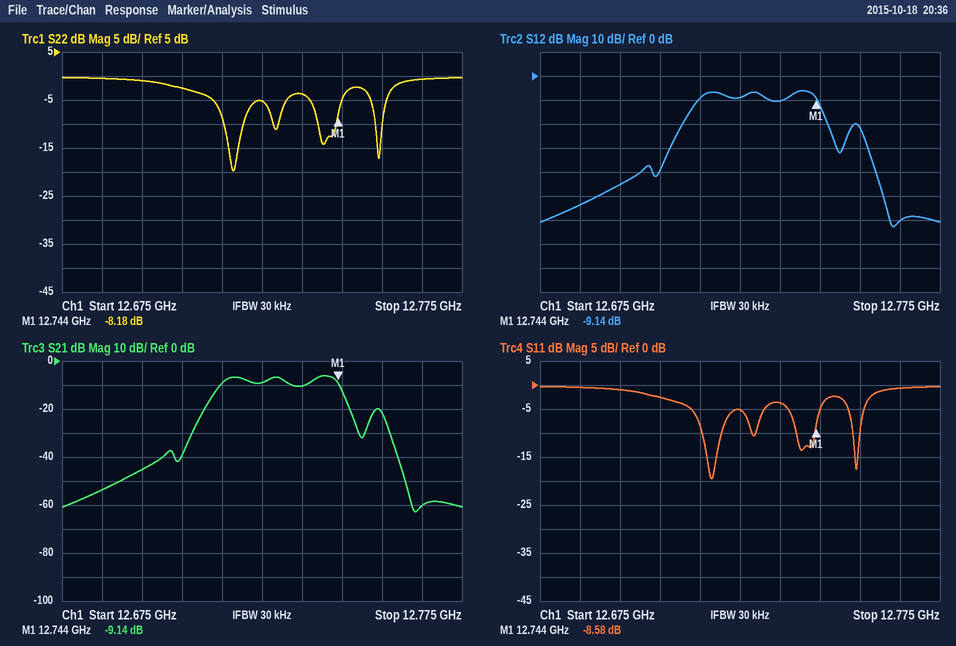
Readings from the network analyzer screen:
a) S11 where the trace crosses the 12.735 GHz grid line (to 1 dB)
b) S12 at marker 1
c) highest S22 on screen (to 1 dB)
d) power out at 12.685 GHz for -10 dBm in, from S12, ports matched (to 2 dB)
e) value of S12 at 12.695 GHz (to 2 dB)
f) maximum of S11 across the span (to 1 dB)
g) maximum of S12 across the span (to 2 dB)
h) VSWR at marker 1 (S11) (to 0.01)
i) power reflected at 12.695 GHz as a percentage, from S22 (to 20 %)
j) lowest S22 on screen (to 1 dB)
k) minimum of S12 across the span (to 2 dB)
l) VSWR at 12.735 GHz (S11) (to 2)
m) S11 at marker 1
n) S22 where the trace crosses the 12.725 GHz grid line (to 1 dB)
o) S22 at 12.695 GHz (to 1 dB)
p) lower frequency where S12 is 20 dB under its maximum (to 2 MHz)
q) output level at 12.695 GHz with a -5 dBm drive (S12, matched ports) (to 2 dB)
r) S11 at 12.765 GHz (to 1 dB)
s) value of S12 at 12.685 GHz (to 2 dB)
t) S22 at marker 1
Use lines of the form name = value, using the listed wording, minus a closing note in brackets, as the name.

S11 where the trace crosses the 12.735 GHz grid line = -4 dB
S12 at marker 1 = -9.14 dB
highest S22 on screen = 0 dB
power out at 12.685 GHz for -10 dBm in, from S12, ports matched = -64 dBm
value of S12 at 12.695 GHz = -46 dB
maximum of S11 across the span = 0 dB
maximum of S12 across the span = -6 dB
VSWR at marker 1 (S11) = 2.19
power reflected at 12.695 GHz as a percentage, from S22 = 80 %
lowest S22 on screen = -20 dB
minimum of S12 across the span = -62 dB
VSWR at 12.735 GHz (S11) = 4
S11 at marker 1 = -8.58 dB
S22 where the trace crosses the 12.725 GHz grid line = -5 dB
S22 at 12.695 GHz = -1 dB
lower frequency where S12 is 20 dB under its maximum = 12.708 GHz
output level at 12.695 GHz with a -5 dBm drive (S12, matched ports) = -50 dBm
S11 at 12.765 GHz = -1 dB
value of S12 at 12.685 GHz = -54 dB
S22 at marker 1 = -8.18 dB
